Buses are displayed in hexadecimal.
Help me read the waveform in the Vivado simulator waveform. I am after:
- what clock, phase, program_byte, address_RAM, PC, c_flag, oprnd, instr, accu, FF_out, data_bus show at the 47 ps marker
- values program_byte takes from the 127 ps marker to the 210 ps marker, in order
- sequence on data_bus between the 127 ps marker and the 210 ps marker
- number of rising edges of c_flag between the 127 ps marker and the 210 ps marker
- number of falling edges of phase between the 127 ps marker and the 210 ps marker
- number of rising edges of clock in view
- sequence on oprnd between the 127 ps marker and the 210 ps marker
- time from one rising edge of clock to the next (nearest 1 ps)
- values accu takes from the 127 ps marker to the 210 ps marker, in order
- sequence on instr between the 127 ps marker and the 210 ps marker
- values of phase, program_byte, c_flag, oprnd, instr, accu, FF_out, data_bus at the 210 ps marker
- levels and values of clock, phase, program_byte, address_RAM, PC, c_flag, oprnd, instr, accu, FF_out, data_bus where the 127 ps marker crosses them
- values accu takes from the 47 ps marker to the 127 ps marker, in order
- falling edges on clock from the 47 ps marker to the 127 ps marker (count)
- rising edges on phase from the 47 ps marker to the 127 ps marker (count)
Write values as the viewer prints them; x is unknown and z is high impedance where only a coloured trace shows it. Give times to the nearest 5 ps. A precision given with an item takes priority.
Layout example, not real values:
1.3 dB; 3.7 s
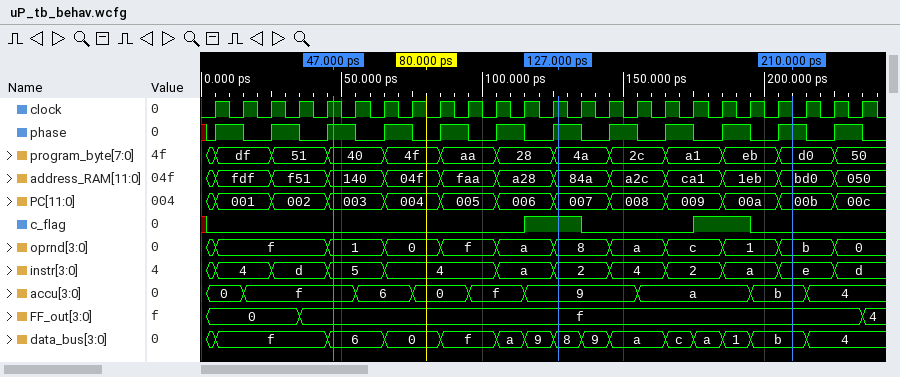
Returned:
clock=1, phase=1, program_byte=40, address_RAM=140, PC=003, c_flag=0, oprnd=1, instr=5, accu=f, FF_out=f, data_bus=6; 4a, 2c, a1, eb, d0; 8, 9, a, c, a, 1, b; 1; 4; 24; 8, a, c, 1, b; 10 ps; 9, a, b; 2, 4, 2, a, e; phase=1, program_byte=d0, c_flag=0, oprnd=b, instr=e, accu=b, FF_out=f, data_bus=b; clock=1, phase=1, program_byte=4a, address_RAM=84a, PC=007, c_flag=1, oprnd=8, instr=2, accu=9, FF_out=f, data_bus=8; f, 6, 0, f, 9; 8; 4
